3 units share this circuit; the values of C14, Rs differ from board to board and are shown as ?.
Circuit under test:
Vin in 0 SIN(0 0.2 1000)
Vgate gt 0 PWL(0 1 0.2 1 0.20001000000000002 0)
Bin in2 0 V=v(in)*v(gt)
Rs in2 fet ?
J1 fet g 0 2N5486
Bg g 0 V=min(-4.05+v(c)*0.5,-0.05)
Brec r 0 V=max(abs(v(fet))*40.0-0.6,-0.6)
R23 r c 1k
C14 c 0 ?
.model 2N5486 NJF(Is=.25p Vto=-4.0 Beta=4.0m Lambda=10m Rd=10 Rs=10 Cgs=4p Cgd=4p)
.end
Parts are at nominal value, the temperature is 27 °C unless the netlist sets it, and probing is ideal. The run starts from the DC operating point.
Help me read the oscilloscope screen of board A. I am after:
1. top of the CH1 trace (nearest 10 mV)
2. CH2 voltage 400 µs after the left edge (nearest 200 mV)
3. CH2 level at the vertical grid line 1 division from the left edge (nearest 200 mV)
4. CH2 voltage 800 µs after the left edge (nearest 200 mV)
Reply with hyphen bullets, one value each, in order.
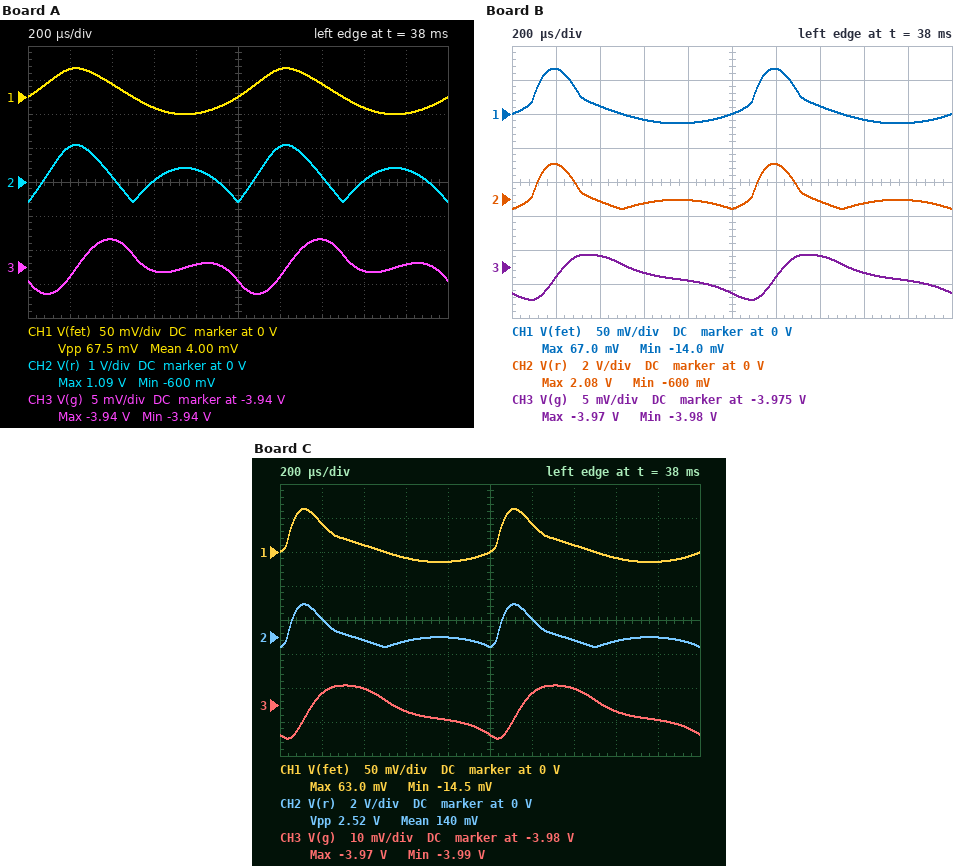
- 40 mV
- 200 mV
- 1.0 V
- 400 mV
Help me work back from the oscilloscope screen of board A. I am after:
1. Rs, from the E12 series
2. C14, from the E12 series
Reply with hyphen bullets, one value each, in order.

- 12 kΩ
- 10 µF
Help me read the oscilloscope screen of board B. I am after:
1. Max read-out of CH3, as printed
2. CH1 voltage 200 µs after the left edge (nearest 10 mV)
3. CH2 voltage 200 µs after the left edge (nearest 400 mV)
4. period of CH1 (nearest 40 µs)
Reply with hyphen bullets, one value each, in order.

- -3.97 V
- 70 mV
- 2.0 V
- 1.00 ms
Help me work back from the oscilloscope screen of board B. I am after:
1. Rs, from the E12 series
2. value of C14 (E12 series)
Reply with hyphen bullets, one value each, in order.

- 56 kΩ
- 22 µF
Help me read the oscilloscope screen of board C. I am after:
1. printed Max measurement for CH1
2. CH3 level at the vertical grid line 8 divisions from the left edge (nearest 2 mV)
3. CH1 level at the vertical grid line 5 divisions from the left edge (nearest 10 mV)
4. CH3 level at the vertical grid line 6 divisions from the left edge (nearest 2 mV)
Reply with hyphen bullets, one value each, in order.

- 63.0 mV
- -3.982 V
- 0 V
- -3.976 V
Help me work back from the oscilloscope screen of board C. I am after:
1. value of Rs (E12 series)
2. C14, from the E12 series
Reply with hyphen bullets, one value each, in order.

- 68 kΩ
- 8.2 µF
